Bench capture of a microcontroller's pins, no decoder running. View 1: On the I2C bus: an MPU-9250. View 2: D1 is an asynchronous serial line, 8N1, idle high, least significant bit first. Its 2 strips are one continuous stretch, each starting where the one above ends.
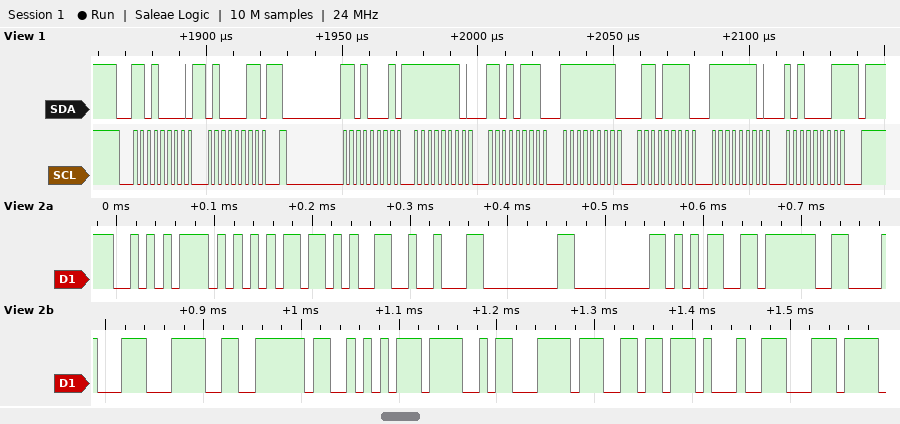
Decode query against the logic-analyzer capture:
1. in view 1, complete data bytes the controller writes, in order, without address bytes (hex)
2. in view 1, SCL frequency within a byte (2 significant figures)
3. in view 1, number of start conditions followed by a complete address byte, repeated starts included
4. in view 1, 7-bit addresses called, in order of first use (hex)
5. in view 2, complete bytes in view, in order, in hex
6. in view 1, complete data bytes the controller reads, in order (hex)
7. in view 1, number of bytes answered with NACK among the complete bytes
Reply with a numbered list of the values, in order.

1. 43
2. 400 kHz
3. 2
4. 0x68
5. AA 55 2B 12 00 00 35 3F 88 3C 7E AA 4F BC B6 91 DC
6. FE D7 FF 6F FE A1
7. 1
